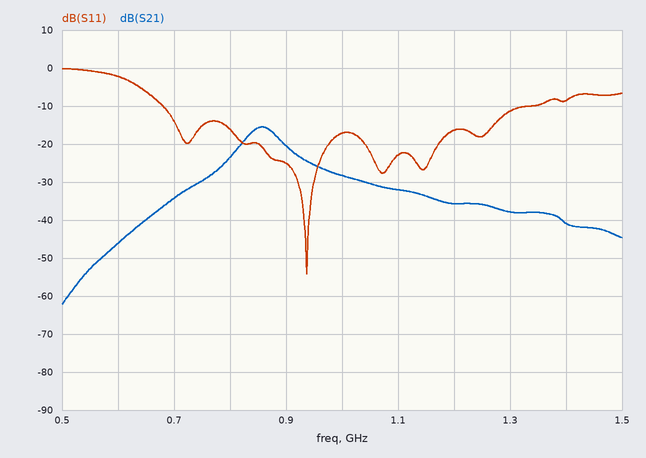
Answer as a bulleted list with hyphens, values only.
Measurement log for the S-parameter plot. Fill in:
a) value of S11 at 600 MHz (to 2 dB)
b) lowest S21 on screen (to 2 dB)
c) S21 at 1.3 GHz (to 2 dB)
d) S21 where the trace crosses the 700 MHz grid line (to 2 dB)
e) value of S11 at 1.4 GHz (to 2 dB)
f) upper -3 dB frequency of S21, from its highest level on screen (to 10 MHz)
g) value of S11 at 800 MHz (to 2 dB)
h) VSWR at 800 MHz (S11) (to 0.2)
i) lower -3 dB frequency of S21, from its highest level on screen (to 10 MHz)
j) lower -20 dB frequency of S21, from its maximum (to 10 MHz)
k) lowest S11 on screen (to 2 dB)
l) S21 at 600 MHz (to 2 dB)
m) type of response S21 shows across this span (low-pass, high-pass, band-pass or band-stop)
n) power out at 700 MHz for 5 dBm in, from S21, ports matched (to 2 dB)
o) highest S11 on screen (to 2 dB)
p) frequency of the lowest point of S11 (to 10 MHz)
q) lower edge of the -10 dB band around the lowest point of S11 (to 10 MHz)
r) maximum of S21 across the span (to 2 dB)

- -2 dB
- -62 dB
- -38 dB
- -34 dB
- -8 dB
- 890 MHz
- -16 dB
- 1.4
- 830 MHz
- 690 MHz
- -54 dB
- -46 dB
- band-pass
- -30 dBm
- 0 dB
- 940 MHz
- 680 MHz
- -16 dB
